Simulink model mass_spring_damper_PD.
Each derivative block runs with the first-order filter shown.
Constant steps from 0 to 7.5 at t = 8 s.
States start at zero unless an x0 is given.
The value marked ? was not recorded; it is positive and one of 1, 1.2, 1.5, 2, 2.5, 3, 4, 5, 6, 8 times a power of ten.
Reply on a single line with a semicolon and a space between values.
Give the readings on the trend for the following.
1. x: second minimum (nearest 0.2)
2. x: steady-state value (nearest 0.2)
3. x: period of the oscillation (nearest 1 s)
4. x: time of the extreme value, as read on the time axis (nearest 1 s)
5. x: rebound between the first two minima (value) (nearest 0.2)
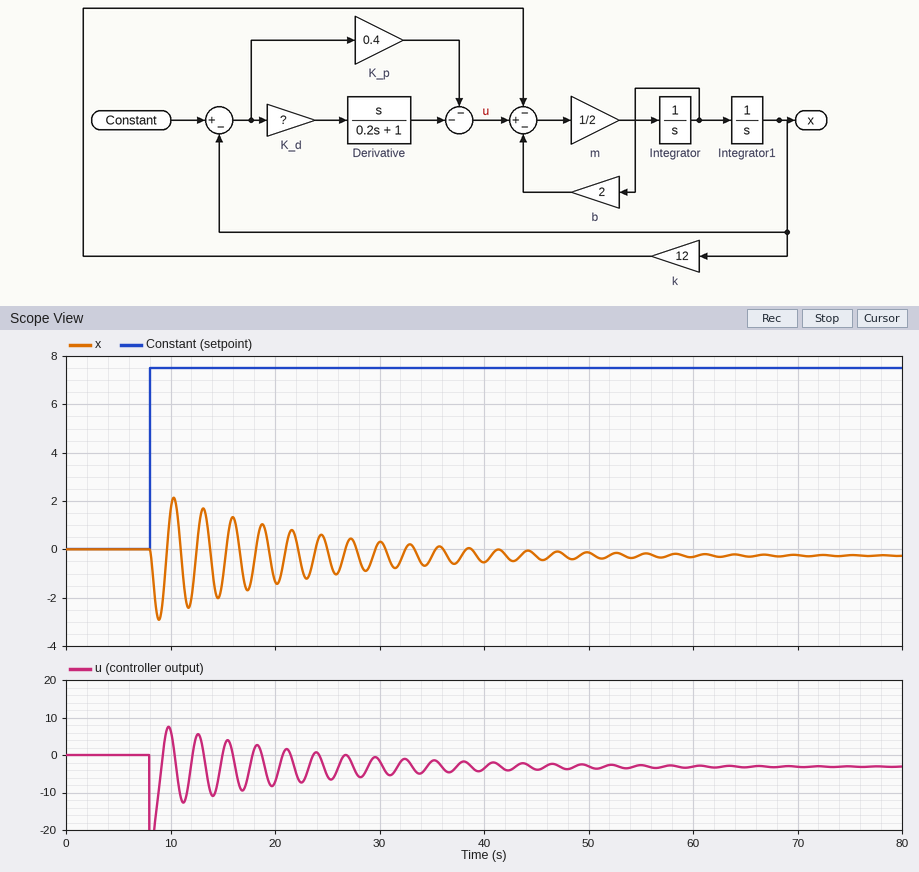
-2.4; -0.2; 3 s; 9 s; 2.2
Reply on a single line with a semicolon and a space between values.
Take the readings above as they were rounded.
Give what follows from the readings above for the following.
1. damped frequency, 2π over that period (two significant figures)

2.1 rad/s
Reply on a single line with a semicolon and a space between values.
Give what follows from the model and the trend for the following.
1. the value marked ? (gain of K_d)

2
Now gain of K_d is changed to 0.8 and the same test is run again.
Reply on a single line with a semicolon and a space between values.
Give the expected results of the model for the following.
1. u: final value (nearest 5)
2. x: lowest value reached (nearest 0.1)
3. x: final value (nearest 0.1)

-5; -1.2; -0.3
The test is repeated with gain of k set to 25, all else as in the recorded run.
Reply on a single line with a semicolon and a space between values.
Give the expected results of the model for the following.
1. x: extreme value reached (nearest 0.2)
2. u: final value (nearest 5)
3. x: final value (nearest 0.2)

-1.8; -5; -0.2
